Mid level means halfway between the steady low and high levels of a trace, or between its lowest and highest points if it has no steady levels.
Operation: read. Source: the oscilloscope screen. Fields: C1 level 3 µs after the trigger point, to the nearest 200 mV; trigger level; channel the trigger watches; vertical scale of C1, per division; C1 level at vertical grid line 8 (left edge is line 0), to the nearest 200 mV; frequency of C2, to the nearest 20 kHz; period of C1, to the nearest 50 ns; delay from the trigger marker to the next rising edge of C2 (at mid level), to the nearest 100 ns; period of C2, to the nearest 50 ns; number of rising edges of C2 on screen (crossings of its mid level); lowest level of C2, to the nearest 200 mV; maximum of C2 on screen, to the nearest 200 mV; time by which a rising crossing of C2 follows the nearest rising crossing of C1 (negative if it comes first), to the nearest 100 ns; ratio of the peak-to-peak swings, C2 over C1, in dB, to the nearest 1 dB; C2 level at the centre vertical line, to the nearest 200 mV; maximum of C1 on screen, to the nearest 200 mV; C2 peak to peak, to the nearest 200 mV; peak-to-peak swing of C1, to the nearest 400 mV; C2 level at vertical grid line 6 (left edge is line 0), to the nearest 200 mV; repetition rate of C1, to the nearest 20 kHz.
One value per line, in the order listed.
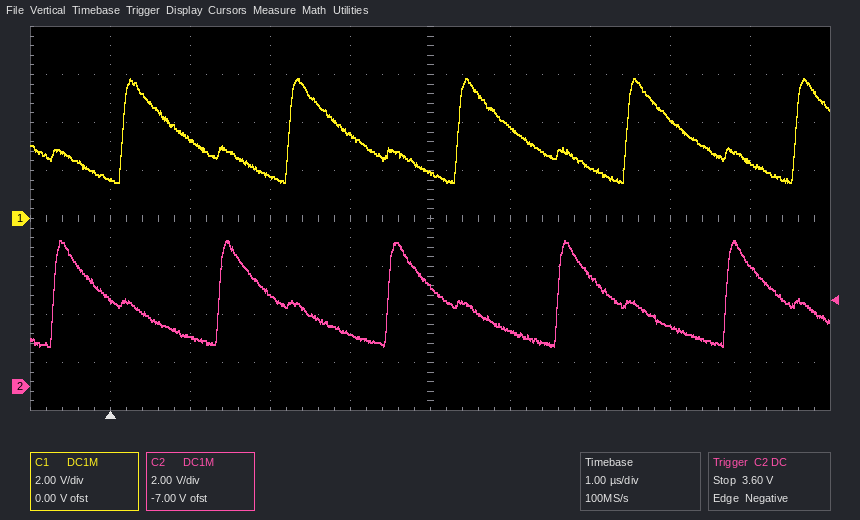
3.4 V
3.60 V
C2
2 V
4.2 V
480 kHz
2.10 µs
1.4 µs
2.10 µs
5
1.6 V
6.0 V
-900 ns
0 dB
4.2 V
5.8 V
4.4 V
4.4 V
2.4 V
480 kHz
